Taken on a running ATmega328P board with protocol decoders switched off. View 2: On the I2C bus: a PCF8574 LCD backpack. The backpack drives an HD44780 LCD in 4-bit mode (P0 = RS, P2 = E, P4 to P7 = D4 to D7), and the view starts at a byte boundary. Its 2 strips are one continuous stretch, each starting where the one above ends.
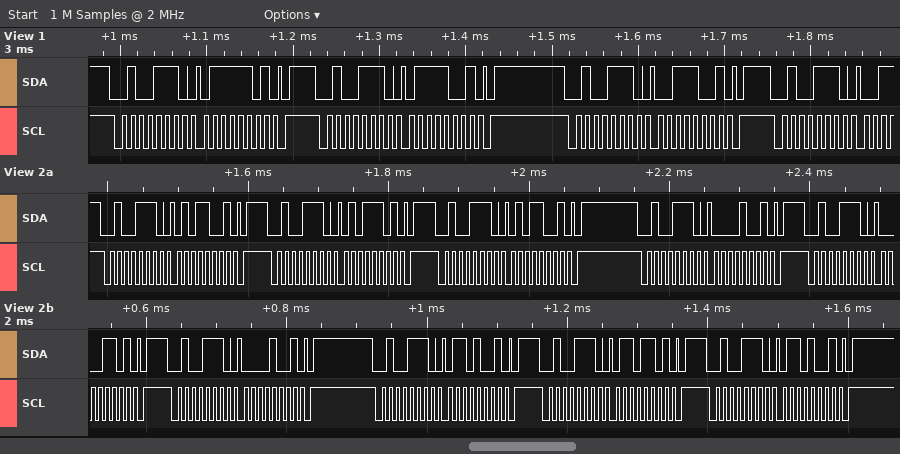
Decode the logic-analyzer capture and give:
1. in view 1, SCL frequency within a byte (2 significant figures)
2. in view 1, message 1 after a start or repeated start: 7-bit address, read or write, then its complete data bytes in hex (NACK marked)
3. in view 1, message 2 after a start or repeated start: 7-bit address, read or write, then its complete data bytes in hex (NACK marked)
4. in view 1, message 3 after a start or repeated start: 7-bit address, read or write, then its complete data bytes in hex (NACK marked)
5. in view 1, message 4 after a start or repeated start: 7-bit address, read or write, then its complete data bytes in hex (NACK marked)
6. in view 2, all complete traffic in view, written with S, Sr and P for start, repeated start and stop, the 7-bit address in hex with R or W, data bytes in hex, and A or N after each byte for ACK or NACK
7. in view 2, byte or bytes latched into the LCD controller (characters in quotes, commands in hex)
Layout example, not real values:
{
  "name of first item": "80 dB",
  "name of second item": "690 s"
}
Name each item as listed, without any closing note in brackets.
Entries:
{
  "in view 1, SCL frequency within a byte": "100 kHz",
  "in view 1, message 1 after a start or repeated start: 7-bit address, read or write, then its complete data bytes in hex": "0x27 write: 7D",
  "in view 1, message 2 after a start or repeated start: 7-bit address, read or write, then its complete data bytes in hex": "0x27 write: 79",
  "in view 1, message 3 after a start or repeated start: 7-bit address, read or write, then its complete data bytes in hex": "0x27 write: 39",
  "in view 1, message 4 after a start or repeated start: 7-bit address, read or write, then its complete data bytes in hex": "0x27 write",
  "in view 2, all complete traffic in view, written with S, Sr and P for start, repeated start and stop, the 7-bit address in hex with R or W, data bytes in hex, and A or N after each byte for ACK or NACK": "S 27W A 59 A P S 27W A 5D A P S 27W A 59 A P S 27W A 09 A P S 27W A 0D A P S 27W A 09 A P S 27W A 69 A P S 27W A 6D A P S 27W A 69 A P",
  "in view 2, byte or bytes latched into the LCD controller": "'P'"
}
